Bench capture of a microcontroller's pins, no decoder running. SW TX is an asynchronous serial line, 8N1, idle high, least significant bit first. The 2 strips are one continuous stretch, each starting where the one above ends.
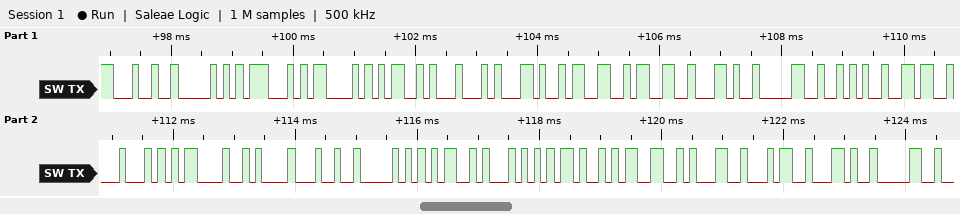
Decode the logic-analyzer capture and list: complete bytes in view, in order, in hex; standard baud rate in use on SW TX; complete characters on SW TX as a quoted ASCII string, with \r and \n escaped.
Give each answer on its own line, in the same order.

24 50 47 43 4D 44 2C 33 33 2C 30 2A 36 44 0D 0A 24 50 4D 54 4B 33 31 34 2C 30
9600 baud
"$PGCMD,33,0*6D\r\n$PMTK314,0"
